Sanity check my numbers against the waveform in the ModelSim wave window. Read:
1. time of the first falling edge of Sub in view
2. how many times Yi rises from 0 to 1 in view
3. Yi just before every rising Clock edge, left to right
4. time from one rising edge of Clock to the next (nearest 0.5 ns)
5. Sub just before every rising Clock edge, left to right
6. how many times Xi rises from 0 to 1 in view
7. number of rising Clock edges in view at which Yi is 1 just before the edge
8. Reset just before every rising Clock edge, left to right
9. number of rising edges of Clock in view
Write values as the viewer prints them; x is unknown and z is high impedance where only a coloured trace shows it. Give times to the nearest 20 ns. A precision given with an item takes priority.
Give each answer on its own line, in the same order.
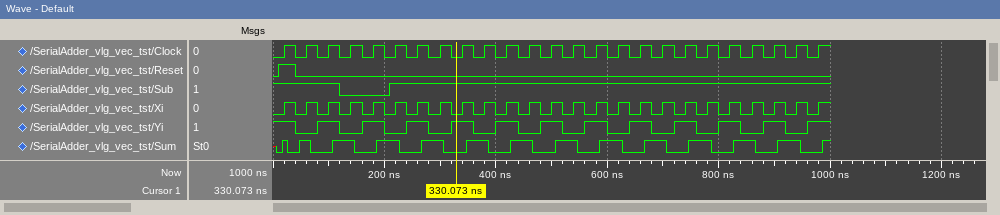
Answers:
120 ns
12
1 0 1 0 1 0 1 0 1 0 1 0 1 0 1 0 1 0 1 0 1 0 1 0 1
40 ns
1 1 1 0 0 1 1 1 1 1 1 1 1 1 1 1 1 1 1 1 1 1 1 1 1
25
13
1 0 0 0 0 0 0 0 0 0 0 0 0 0 0 0 0 0 0 0 0 0 0 0 0
25
